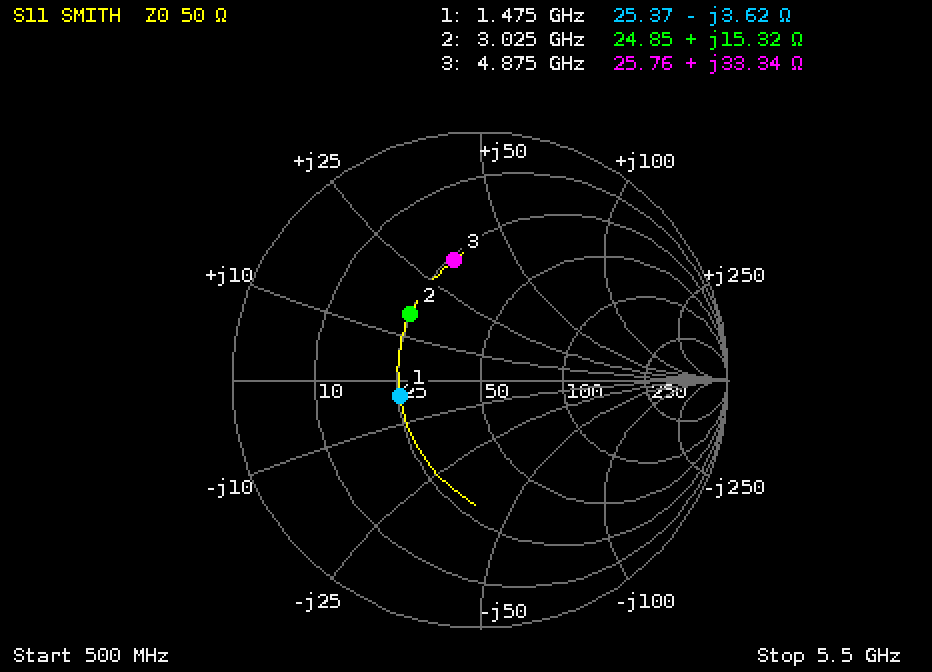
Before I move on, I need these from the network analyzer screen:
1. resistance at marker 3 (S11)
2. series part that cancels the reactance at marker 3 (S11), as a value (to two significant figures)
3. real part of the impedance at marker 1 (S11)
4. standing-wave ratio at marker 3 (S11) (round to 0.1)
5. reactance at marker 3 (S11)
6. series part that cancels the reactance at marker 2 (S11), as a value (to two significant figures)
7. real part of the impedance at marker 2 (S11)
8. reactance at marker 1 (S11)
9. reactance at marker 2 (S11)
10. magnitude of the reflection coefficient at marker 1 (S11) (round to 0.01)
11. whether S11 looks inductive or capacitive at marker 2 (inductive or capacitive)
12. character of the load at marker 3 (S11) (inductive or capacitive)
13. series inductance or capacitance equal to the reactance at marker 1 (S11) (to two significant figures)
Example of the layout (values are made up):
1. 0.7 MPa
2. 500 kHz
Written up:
1. 25.76 Ω
2. 980 fF
3. 25.37 Ω
4. 3.0
5. +33.34 Ω
6. 3.4 pF
7. 24.85 Ω
8. -3.62 Ω
9. +15.32 Ω
10. 0.33
11. inductive
12. inductive
13. 30 pF
